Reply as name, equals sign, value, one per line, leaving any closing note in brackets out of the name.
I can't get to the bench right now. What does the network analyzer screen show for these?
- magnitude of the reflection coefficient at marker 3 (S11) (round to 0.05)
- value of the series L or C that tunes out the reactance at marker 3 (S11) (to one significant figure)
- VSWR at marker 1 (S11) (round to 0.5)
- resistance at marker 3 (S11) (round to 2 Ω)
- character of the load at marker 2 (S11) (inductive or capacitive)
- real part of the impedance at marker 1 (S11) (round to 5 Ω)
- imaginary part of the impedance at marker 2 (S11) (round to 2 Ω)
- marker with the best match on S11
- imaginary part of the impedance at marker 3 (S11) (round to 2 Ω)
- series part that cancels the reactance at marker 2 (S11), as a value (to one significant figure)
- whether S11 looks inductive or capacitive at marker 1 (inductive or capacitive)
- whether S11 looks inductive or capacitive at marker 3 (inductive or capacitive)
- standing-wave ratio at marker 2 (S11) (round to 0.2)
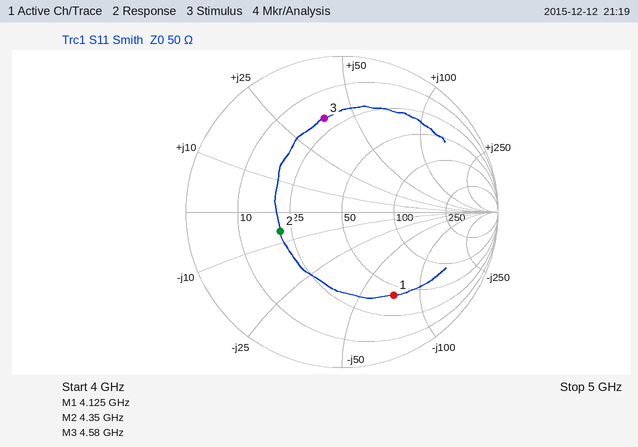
magnitude of the reflection coefficient at marker 3 (S11) = 0.60
value of the series L or C that tunes out the reactance at marker 3 (S11) = 900 fF
VSWR at marker 1 (S11) = 4.5
resistance at marker 3 (S11) = 20 Ω
character of the load at marker 2 (S11) = capacitive
real part of the impedance at marker 1 (S11) = 40 Ω
imaginary part of the impedance at marker 2 (S11) = -6 Ω
marker with the best match on S11 = marker 2
imaginary part of the impedance at marker 3 (S11) = +38 Ω
series part that cancels the reactance at marker 2 (S11), as a value = 200 pH
whether S11 looks inductive or capacitive at marker 1 = capacitive
whether S11 looks inductive or capacitive at marker 3 = inductive
standing-wave ratio at marker 2 (S11) = 2.4
